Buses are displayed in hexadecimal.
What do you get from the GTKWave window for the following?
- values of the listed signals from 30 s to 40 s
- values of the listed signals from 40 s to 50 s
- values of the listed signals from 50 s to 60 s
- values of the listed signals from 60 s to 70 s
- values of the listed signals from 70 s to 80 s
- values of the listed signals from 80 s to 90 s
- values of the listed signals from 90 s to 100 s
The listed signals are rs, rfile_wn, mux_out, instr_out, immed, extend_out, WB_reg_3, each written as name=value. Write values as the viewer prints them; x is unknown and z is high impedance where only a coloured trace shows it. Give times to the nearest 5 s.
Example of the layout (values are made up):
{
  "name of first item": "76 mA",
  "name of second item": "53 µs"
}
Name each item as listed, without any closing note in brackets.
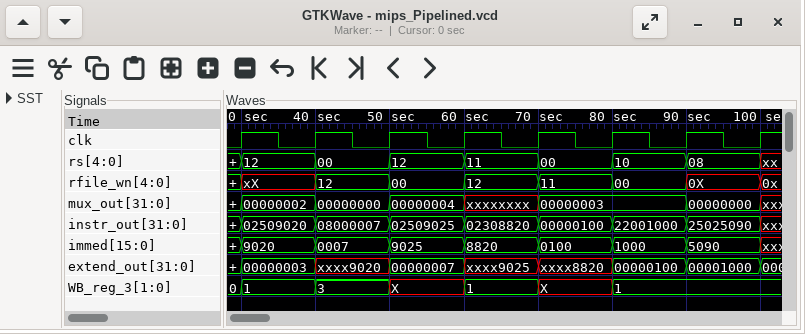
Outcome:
{
  "values of the listed signals from 30 s to 40 s": "rs=12, rfile_wn=xX, mux_out=00000002, instr_out=02509020, immed=9020, extend_out=00000003, WB_reg_3=1",
  "values of the listed signals from 40 s to 50 s": "rs=00, rfile_wn=12, mux_out=00000000, instr_out=08000007, immed=0007, extend_out=xxxx9020, WB_reg_3=3",
  "values of the listed signals from 50 s to 60 s": "rs=12, rfile_wn=00, mux_out=00000004, instr_out=02509025, immed=9025, extend_out=00000007, WB_reg_3=X",
  "values of the listed signals from 60 s to 70 s": "rs=11, rfile_wn=12, mux_out=xxxxxxxx, instr_out=02308820, immed=8820, extend_out=xxxx9025, WB_reg_3=1",
  "values of the listed signals from 70 s to 80 s": "rs=00, rfile_wn=11, mux_out=00000003, instr_out=00000100, immed=0100, extend_out=xxxx8820, WB_reg_3=X",
  "values of the listed signals from 80 s to 90 s": "rs=10, rfile_wn=00, mux_out=00000003, instr_out=22001000, immed=1000, extend_out=00000100, WB_reg_3=1",
  "values of the listed signals from 90 s to 100 s": "rs=08, rfile_wn=0X, mux_out=00000000, instr_out=25025090, immed=5090, extend_out=00001000, WB_reg_3=1"
}
